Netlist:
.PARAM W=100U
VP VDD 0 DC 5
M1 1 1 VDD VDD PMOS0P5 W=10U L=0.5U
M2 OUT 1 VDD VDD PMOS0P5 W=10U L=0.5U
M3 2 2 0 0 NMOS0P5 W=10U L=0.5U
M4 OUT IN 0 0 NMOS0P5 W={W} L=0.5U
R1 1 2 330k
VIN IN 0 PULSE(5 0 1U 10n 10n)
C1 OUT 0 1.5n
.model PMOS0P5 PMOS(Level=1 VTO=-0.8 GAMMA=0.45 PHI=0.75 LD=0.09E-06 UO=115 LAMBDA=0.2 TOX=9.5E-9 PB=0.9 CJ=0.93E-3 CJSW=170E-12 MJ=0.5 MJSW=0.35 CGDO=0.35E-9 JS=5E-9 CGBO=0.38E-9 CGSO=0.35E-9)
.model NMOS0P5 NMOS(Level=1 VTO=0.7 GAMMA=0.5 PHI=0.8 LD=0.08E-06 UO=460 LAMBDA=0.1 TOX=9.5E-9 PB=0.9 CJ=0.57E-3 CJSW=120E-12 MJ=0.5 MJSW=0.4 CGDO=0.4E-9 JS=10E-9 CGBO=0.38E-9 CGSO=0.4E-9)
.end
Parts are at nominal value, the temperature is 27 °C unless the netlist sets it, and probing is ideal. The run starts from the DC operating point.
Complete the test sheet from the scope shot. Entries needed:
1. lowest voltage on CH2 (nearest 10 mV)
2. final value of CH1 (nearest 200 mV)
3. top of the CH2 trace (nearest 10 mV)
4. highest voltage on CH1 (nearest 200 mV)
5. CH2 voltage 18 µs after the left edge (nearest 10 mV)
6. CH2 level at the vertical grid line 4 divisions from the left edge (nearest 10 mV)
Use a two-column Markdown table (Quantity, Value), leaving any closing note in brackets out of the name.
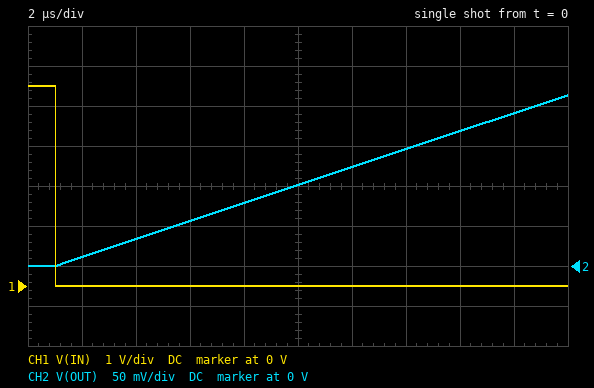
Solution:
| Quantity | Value |
|---|---|
| lowest voltage on CH2 | 0 V |
| final value of CH1 | 0 V |
| top of the CH2 trace | 210 mV |
| highest voltage on CH1 | 5.0 V |
| CH2 voltage 18 µs after the left edge | 190 mV |
| CH2 level at the vertical grid line 4 divisions from the left edge | 80 mV |
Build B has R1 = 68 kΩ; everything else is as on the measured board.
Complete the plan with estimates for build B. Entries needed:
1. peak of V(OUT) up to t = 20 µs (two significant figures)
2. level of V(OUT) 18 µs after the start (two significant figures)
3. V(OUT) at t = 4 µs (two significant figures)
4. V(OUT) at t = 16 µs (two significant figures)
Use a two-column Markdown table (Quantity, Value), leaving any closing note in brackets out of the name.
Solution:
| Quantity | Value |
|---|---|
| peak of V(OUT) up to t = 20 µs | 920 mV |
| level of V(OUT) 18 µs after the start | 830 mV |
| V(OUT) at t = 4 µs | 150 mV |
| V(OUT) at t = 16 µs | 730 mV |
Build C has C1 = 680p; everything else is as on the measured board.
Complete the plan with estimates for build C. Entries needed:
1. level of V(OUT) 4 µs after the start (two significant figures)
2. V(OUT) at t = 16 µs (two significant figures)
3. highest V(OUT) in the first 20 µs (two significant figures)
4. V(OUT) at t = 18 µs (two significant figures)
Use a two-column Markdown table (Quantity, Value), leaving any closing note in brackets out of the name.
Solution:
| Quantity | Value |
|---|---|
| level of V(OUT) 4 µs after the start | 74 mV |
| V(OUT) at t = 16 µs | 370 mV |
| highest V(OUT) in the first 20 µs | 460 mV |
| V(OUT) at t = 18 µs | 420 mV |
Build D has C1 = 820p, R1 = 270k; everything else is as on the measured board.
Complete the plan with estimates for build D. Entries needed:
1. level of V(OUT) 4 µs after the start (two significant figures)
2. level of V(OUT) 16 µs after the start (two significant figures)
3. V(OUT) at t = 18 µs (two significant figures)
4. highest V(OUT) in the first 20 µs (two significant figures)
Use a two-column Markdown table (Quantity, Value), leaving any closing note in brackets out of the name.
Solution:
| Quantity | Value |
|---|---|
| level of V(OUT) 4 µs after the start | 75 mV |
| level of V(OUT) 16 µs after the start | 370 mV |
| V(OUT) at t = 18 µs | 420 mV |
| highest V(OUT) in the first 20 µs | 470 mV |
